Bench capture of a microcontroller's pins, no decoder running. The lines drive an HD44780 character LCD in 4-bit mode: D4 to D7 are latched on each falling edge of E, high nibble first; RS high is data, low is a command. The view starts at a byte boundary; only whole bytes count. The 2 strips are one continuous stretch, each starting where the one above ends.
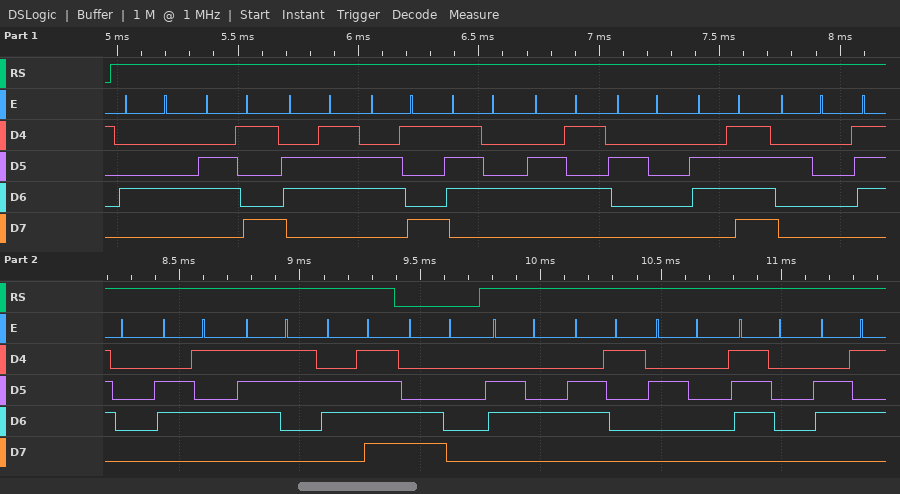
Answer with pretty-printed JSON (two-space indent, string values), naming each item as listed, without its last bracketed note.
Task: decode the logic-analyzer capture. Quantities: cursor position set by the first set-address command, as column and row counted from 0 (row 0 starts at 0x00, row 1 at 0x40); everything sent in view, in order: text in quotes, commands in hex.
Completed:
{
  "cursor position set by the first set-address command, as column and row counted from 0": "column 0, row 1",
  "everything sent in view, in order: text in quotes, commands in hex": "\"Digite o peso\" 0xC0 \"da pe\""
}
